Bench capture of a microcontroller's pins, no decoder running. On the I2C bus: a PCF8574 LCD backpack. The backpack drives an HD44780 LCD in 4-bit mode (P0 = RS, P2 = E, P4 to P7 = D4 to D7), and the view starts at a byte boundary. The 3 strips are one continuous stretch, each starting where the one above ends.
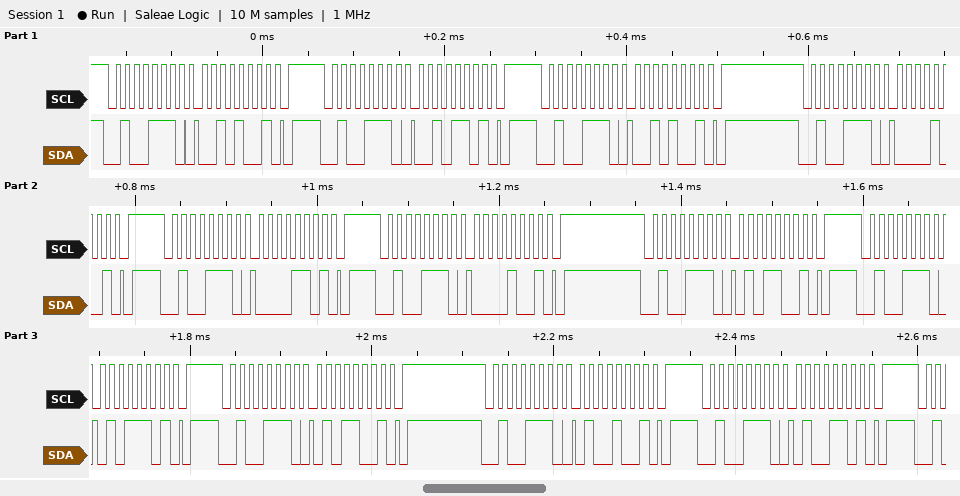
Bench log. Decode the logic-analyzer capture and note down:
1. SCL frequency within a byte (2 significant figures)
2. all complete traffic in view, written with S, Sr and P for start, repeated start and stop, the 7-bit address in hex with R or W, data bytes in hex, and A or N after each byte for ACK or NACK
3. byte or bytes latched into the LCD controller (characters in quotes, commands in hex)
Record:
100 kHz
S 27W A 29 A P S 27W A 2D A P S 27W A 29 A P S 27W A 09 A P S 27W A 0D A P S 27W A 09 A P S 27W A 59 A P S 27W A 5D A P S 27W A 59 A P S 27W A 49 A P S 27W A 4D A P
' '
